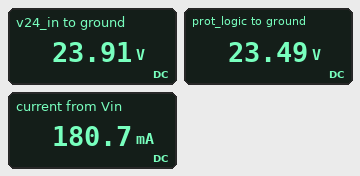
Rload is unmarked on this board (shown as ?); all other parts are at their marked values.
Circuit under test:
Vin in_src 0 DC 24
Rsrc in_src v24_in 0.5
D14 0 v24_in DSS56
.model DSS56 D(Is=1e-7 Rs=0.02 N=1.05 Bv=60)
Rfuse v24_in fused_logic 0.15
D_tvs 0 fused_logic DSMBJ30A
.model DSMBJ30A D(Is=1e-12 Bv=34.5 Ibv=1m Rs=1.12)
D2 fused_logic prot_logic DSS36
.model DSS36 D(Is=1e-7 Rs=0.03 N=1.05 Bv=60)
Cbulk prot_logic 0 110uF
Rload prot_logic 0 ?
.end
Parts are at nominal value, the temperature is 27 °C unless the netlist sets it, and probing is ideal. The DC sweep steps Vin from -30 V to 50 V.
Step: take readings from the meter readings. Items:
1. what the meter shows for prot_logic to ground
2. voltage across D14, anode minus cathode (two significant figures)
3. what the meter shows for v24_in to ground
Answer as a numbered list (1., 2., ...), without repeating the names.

1. 23.49 V
2. -24 V
3. 23.91 V
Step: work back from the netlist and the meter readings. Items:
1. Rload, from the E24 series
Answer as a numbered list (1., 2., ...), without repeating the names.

1. 130 Ω
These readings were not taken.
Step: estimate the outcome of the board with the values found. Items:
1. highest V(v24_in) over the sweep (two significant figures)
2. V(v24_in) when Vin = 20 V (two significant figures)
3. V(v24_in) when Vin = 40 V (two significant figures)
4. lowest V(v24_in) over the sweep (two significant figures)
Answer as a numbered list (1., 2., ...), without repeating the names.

1. 46 V
2. 20 V
3. 38 V
4. -1.7 V
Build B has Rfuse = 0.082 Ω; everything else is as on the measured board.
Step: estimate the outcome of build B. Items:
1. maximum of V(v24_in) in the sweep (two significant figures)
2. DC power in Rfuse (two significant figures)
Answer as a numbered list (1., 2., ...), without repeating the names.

1. 45 V
2. 2.7 mW
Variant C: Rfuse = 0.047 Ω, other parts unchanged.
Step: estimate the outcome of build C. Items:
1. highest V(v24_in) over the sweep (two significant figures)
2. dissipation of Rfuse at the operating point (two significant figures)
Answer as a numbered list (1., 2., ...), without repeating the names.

1. 45 V
2. 1.5 mW
